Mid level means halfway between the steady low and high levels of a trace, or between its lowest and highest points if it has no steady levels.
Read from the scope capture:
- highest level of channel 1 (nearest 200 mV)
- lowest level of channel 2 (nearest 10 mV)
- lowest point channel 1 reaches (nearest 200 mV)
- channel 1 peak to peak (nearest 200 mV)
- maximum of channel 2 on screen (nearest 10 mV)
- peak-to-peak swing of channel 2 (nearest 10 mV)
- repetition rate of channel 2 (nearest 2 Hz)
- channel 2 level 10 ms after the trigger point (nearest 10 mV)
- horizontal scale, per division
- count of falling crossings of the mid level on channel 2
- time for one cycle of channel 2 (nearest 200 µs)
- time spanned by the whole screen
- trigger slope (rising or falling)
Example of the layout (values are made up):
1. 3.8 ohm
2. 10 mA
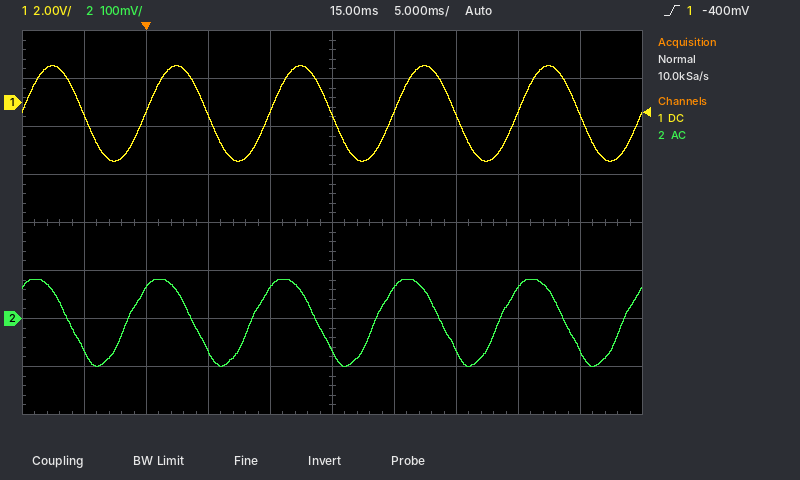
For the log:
1. 1.6 V
2. -100 mV
3. -2.4 V
4. 4.0 V
5. 80 mV
6. 180 mV
7. 100 Hz
8. 60 mV
9. 5 ms
10. 5
11. 10.0 ms
12. 50 ms
13. rising
